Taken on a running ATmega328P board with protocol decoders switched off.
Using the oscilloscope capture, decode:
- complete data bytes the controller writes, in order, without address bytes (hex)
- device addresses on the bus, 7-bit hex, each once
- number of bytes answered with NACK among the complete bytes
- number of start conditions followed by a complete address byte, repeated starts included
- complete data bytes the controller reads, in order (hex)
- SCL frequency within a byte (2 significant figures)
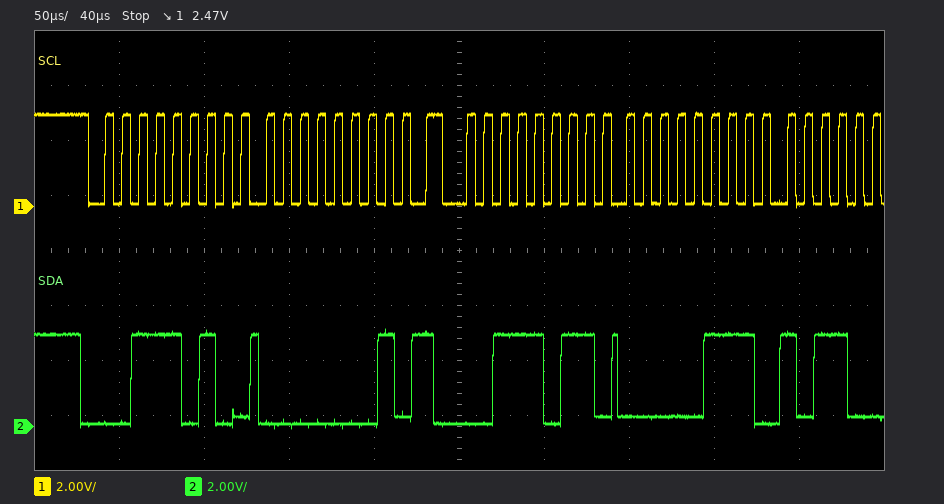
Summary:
01
0x1D
0
2
07
100 kHz
